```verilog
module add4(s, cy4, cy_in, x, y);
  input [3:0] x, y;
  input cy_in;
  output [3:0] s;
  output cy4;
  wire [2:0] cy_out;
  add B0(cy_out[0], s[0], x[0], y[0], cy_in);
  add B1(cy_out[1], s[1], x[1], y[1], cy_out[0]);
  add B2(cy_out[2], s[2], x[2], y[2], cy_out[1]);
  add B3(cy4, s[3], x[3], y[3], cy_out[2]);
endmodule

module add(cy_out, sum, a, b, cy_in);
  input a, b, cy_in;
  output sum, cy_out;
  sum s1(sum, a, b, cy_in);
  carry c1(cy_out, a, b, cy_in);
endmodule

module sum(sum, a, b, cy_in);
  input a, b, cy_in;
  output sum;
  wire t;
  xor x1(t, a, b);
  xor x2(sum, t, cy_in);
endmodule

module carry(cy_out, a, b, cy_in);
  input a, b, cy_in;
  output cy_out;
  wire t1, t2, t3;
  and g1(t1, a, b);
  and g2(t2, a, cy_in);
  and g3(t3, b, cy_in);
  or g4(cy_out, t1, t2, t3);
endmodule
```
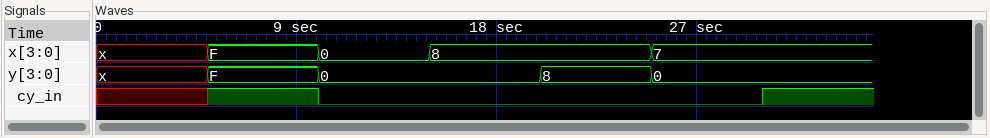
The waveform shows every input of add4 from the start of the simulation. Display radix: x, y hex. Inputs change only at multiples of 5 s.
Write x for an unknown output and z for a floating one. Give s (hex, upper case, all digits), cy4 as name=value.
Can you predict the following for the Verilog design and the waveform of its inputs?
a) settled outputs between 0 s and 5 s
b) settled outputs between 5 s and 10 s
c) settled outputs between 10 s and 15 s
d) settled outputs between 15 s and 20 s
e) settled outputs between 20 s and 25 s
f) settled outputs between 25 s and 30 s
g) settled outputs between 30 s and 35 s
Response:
s=x, cy4=x
s=F, cy4=1
s=0, cy4=0
s=8, cy4=0
s=0, cy4=1
s=7, cy4=0
s=8, cy4=0
